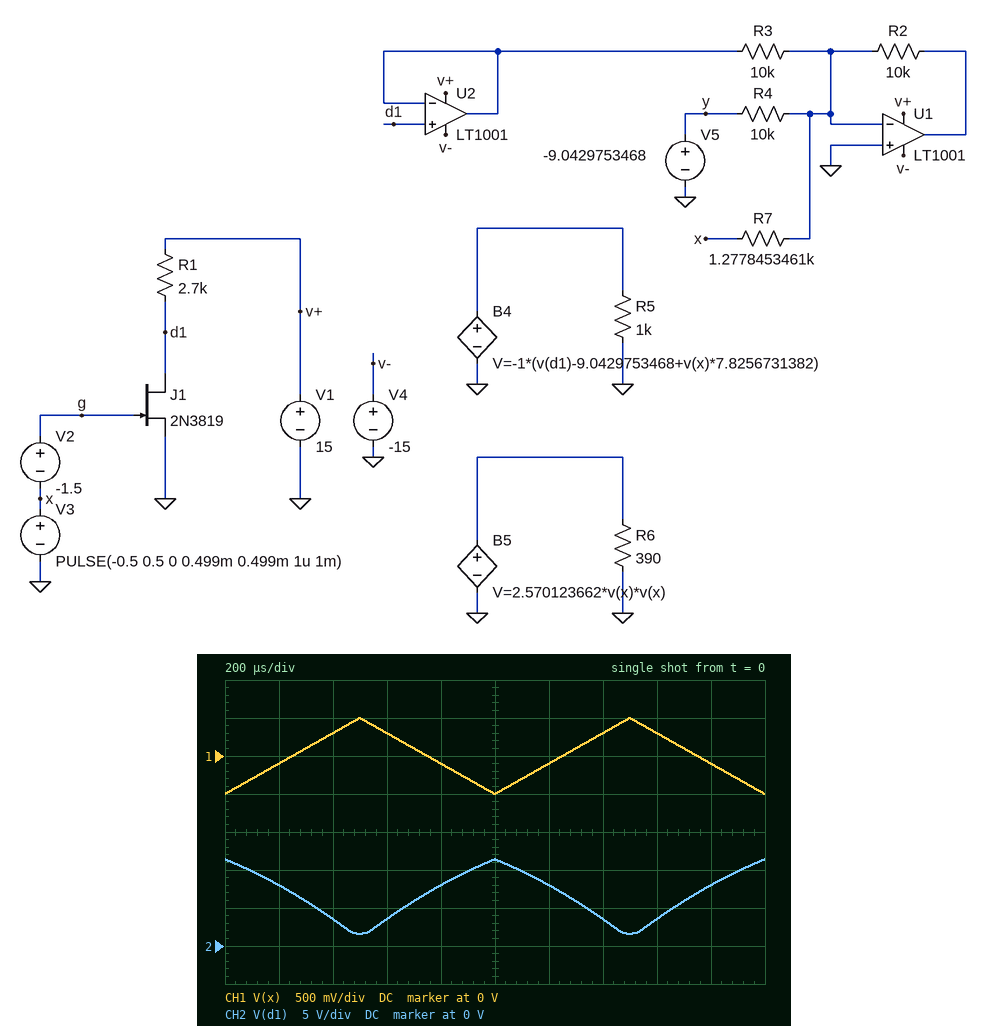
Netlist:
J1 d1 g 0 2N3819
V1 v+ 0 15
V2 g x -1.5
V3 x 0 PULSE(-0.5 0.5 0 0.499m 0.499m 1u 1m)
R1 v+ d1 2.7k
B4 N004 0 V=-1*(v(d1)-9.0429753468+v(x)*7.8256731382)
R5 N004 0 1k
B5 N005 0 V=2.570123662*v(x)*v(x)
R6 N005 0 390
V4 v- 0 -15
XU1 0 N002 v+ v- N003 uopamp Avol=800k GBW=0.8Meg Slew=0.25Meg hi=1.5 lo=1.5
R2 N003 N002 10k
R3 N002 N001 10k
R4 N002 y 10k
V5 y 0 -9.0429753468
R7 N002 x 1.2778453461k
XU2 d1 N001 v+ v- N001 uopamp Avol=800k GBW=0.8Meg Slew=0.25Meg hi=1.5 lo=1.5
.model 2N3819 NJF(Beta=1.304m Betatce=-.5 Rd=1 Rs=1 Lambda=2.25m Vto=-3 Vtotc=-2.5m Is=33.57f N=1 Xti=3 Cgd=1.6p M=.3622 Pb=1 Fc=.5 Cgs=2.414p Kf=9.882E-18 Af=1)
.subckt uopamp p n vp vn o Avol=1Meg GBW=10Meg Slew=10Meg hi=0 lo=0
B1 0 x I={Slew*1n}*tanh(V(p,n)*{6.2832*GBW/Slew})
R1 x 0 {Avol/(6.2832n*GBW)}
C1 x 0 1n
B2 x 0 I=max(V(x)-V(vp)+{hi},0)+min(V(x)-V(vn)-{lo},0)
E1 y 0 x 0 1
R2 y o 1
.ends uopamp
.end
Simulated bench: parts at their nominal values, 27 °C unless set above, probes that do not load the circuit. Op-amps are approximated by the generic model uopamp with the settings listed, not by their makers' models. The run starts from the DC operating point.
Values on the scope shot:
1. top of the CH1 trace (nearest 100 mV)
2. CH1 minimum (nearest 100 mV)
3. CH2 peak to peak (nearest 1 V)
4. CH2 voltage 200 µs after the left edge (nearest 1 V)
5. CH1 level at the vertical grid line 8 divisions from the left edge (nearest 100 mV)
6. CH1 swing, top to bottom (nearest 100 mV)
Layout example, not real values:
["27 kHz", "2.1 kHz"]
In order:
["500 mV", "-500 mV", "10 V", "8 V", "300 mV", "1.0 V"]
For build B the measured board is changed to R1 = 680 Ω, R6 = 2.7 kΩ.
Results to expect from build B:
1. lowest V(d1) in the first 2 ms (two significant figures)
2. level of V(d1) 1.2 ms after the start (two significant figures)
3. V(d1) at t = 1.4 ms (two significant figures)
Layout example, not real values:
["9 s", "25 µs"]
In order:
["11 V", "13 V", "12 V"]
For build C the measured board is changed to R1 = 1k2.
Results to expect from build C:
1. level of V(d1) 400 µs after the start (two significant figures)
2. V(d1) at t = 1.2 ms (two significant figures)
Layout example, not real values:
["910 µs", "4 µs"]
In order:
["9.8 V", "12 V"]
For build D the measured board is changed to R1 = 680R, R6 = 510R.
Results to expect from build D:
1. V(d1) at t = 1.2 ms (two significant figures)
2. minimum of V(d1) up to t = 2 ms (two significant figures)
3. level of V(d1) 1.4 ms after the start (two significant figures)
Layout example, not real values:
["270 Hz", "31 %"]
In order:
["13 V", "11 V", "12 V"]
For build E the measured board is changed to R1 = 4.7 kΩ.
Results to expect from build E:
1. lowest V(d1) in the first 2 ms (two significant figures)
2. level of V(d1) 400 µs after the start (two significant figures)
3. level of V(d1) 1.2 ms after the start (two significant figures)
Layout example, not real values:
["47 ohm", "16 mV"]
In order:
["710 mV", "840 mV", "2.9 V"]
